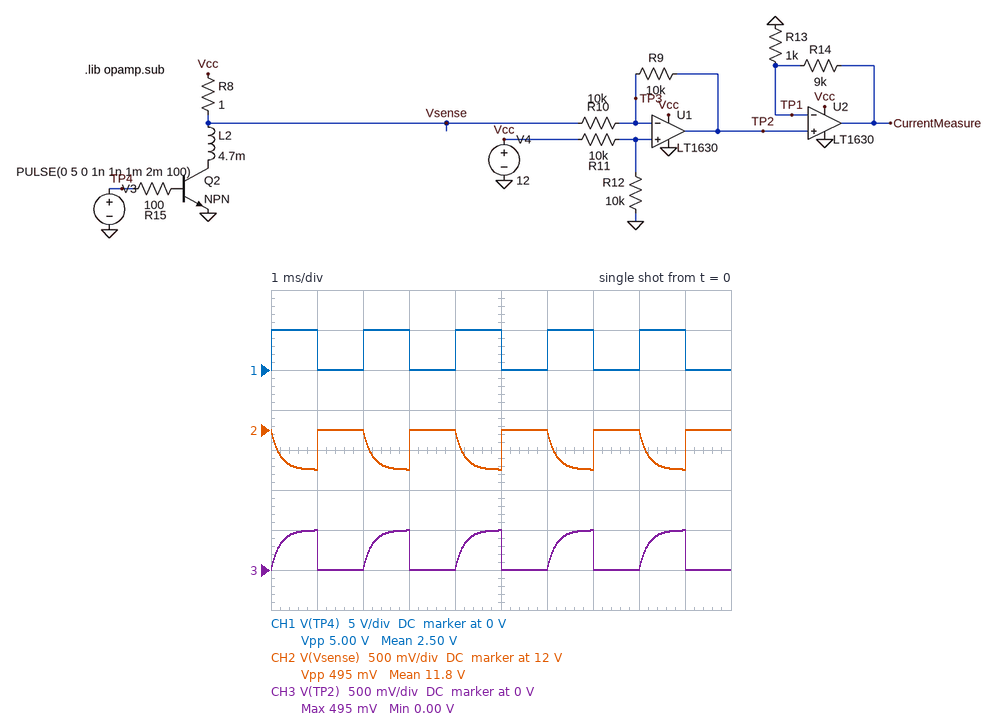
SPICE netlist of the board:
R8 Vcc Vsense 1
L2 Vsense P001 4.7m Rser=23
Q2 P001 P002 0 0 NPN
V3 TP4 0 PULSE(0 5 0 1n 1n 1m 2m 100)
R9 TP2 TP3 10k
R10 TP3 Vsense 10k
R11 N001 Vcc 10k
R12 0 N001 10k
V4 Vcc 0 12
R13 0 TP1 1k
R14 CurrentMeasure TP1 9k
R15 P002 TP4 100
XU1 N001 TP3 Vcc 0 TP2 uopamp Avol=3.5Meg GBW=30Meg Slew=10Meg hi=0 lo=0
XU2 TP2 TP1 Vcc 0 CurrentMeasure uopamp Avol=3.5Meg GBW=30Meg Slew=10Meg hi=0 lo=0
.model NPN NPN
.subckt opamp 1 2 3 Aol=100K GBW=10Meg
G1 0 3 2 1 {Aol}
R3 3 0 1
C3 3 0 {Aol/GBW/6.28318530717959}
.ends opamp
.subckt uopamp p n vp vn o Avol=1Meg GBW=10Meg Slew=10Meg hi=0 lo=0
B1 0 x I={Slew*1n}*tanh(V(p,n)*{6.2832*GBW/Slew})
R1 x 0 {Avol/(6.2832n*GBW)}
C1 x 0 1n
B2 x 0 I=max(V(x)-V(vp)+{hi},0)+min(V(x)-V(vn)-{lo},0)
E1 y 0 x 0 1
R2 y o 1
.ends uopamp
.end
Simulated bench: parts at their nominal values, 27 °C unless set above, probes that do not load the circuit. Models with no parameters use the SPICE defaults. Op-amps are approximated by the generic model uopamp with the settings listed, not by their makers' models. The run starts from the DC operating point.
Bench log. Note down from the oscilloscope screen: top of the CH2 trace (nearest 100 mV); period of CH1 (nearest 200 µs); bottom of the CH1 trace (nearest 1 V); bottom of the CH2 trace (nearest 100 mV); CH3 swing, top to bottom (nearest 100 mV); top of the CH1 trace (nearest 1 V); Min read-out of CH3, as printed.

12.0 V
2.0 ms
0 V
11.5 V
500 mV
5 V
0.00 V
